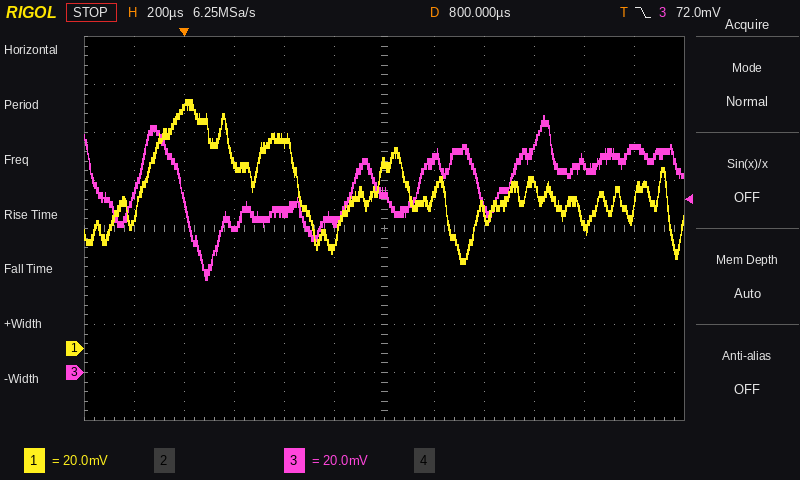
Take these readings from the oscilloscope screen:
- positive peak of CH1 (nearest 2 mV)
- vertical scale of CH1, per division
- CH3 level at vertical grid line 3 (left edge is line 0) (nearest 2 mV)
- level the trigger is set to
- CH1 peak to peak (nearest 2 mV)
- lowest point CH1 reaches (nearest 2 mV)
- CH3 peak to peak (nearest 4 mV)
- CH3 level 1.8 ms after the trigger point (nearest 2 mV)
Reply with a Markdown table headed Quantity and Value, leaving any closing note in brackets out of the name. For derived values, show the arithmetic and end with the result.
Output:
| Quantity | Value |
|---|---|
| positive peak of CH1 | 104 mV |
| vertical scale of CH1, per division | 20 mV |
| CH3 level at vertical grid line 3 (left edge is line 0) | 60 mV |
| level the trigger is set to | 72.0 mV |
| CH1 peak to peak | 104 mV − (36 mV) = 68 mV |
| lowest point CH1 reaches | 36 mV |
| CH3 peak to peak | 68 mV |
| CH3 level 1.8 ms after the trigger point | 94 mV |
